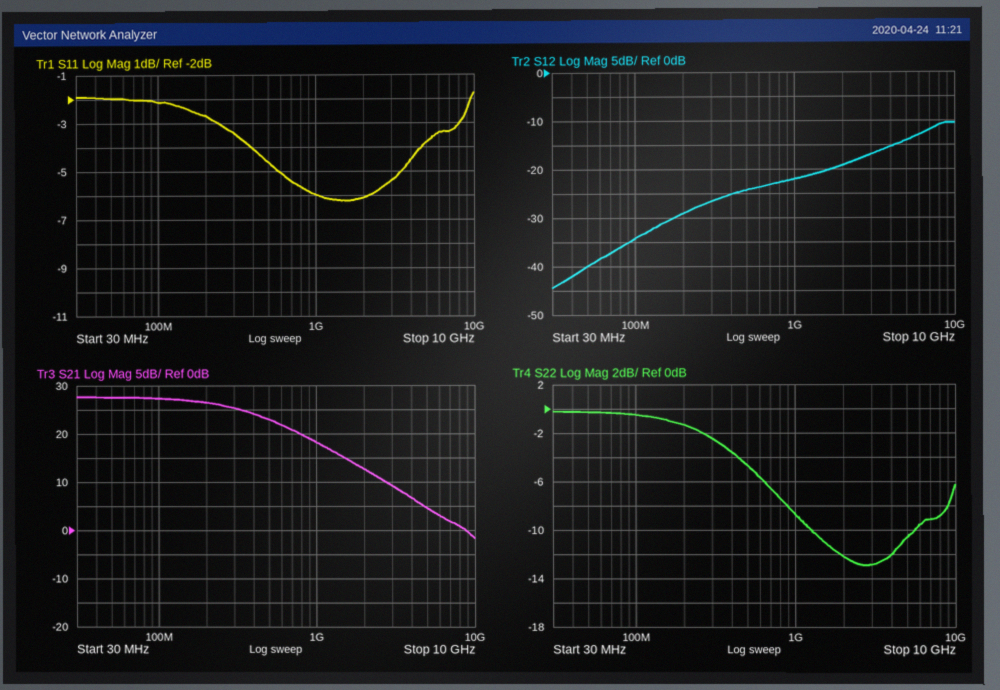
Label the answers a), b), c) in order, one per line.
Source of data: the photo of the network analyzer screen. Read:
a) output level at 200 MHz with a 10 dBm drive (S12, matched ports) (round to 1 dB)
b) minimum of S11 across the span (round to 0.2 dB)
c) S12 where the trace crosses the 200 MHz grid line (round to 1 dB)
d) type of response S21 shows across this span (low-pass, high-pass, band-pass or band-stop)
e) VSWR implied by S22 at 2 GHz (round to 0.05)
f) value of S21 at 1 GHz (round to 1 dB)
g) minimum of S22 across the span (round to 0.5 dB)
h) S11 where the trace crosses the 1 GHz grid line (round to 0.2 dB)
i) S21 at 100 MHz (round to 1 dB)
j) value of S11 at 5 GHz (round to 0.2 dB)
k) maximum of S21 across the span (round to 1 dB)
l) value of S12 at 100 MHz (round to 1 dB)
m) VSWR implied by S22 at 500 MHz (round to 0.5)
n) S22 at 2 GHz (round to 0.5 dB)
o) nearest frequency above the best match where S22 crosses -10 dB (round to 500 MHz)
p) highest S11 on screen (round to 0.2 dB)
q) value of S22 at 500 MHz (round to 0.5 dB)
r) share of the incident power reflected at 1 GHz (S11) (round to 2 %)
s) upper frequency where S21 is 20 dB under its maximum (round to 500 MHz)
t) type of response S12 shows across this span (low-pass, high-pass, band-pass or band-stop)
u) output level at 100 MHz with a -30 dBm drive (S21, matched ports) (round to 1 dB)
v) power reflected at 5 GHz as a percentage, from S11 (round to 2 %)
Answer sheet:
a) -19 dBm
b) -6.2 dB
c) -29 dB
d) low-pass
e) 1.65
f) 18 dB
g) -13.0 dB
h) -6.0 dB
i) 27 dB
j) -3.8 dB
k) 28 dB
l) -34 dB
m) 4.0
n) -12.0 dB
o) 5.5 GHz
p) -1.8 dB
q) -4.5 dB
r) 26 %
s) 3.5 GHz
t) high-pass
u) -3 dBm
v) 42 %
